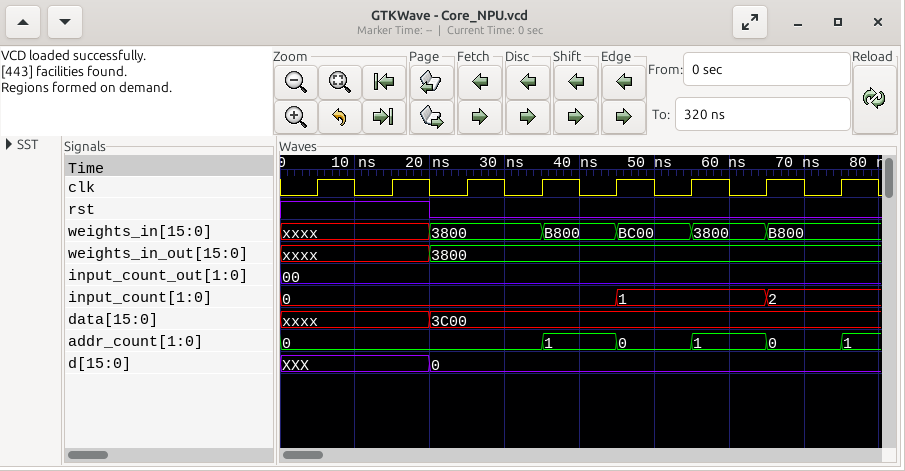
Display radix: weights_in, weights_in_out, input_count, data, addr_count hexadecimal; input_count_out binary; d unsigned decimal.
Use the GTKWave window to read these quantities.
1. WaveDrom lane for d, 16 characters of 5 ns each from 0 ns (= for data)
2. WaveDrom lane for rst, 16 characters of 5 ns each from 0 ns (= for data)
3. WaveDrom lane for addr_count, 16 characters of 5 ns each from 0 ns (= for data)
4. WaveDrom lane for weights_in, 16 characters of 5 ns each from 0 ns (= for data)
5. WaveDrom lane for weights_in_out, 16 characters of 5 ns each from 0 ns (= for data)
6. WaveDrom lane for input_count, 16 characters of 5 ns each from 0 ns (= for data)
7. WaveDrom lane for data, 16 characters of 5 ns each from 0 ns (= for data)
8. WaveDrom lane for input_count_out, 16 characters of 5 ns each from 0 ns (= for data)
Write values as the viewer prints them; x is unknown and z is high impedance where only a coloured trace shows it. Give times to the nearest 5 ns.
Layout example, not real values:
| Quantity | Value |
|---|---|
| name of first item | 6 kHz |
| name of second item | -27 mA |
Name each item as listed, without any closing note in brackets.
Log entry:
| Quantity | Value |
|---|---|
| WaveDrom lane for d, 16 characters of 5 ns each from 0 ns | {name: 'd', wave: 'x...=...........', data: '0'} |
| WaveDrom lane for rst, 16 characters of 5 ns each from 0 ns | {name: 'rst', wave: '1...0...........'} |
| WaveDrom lane for addr_count, 16 characters of 5 ns each from 0 ns | {name: 'addr_count', wave: '=......=.=.=.=.=', data: '0 1 0 1 0 1'} |
| WaveDrom lane for weights_in, 16 characters of 5 ns each from 0 ns | {name: 'weights_in', wave: 'x...=..=.=.=.=..', data: '3800 B800 BC00 3800 B800'} |
| WaveDrom lane for weights_in_out, 16 characters of 5 ns each from 0 ns | {name: 'weights_in_out', wave: 'x...=...........', data: '3800'} |
| WaveDrom lane for input_count, 16 characters of 5 ns each from 0 ns | {name: 'input_count', wave: '=........=...=..', data: '0 1 2'} |
| WaveDrom lane for data, 16 characters of 5 ns each from 0 ns | {name: 'data', wave: 'x...=...........', data: '3C00'} |
| WaveDrom lane for input_count_out, 16 characters of 5 ns each from 0 ns | {name: 'input_count_out', wave: '=...............', data: '00'} |
